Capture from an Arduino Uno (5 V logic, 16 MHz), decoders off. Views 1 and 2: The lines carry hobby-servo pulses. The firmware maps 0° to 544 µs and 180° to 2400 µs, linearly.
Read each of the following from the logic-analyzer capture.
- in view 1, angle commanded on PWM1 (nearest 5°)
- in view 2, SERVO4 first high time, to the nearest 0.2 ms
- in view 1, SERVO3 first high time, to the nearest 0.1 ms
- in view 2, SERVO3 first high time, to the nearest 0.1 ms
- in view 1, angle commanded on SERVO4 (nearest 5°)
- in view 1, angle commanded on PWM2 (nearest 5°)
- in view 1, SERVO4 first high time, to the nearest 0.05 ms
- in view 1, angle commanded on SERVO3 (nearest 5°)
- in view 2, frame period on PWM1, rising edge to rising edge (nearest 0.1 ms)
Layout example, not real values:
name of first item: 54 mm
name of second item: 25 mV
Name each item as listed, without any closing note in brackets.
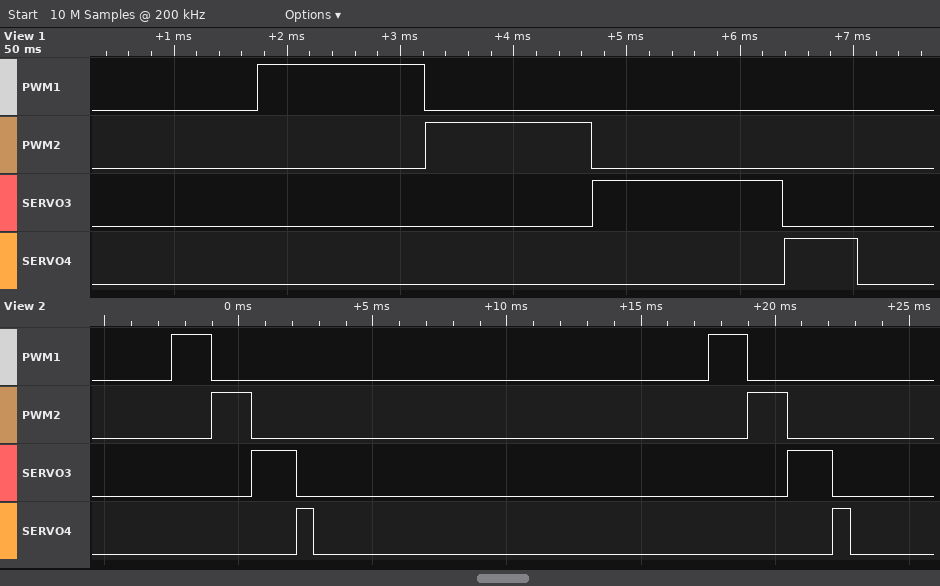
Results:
in view 1, angle commanded on PWM1: 90°
in view 2, SERVO4 first high time, to the nearest 0.2 ms: 0.6 ms
in view 1, SERVO3 first high time, to the nearest 0.1 ms: 1.7 ms
in view 2, SERVO3 first high time, to the nearest 0.1 ms: 1.7 ms
in view 1, angle commanded on SERVO4: 10°
in view 1, angle commanded on PWM2: 90°
in view 1, SERVO4 first high time, to the nearest 0.05 ms: 0.65 ms
in view 1, angle commanded on SERVO3: 110°
in view 2, frame period on PWM1, rising edge to rising edge: 20.0 ms
